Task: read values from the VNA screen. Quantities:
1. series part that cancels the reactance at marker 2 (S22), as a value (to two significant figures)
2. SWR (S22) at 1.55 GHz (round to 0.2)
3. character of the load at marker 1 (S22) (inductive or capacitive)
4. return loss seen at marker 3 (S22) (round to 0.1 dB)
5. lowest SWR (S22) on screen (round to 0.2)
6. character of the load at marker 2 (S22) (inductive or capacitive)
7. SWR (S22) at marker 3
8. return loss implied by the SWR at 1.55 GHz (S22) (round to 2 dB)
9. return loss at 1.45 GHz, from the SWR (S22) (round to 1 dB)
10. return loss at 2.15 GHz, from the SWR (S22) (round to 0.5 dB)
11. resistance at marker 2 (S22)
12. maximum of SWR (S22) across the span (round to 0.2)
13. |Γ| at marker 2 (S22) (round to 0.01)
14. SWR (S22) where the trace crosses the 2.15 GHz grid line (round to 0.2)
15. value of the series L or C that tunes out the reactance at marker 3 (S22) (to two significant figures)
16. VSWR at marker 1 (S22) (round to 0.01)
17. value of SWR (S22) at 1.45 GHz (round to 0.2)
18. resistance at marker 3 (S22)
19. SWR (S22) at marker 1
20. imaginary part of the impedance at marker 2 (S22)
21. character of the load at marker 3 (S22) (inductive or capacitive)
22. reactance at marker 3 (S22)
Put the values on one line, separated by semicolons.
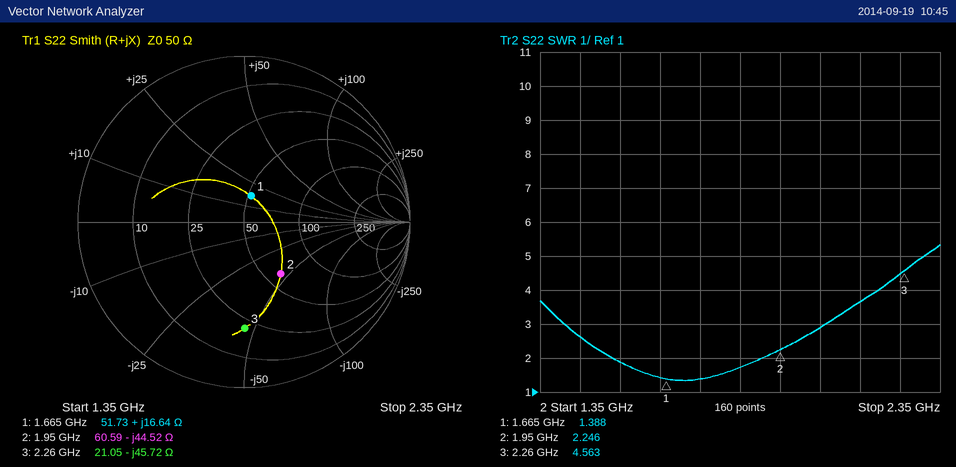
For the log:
3.6 nH; 1.8; inductive; 3.9 dB; 1.4; capacitive; 4.563; 10 dB; 7 dB; 5.0 dB; 60.59 Ω; 5.4; 0.38; 3.6; 3.2 nH; 1.39; 2.6; 21.05 Ω; 1.388; -44.52 Ω; capacitive; -45.72 Ω
